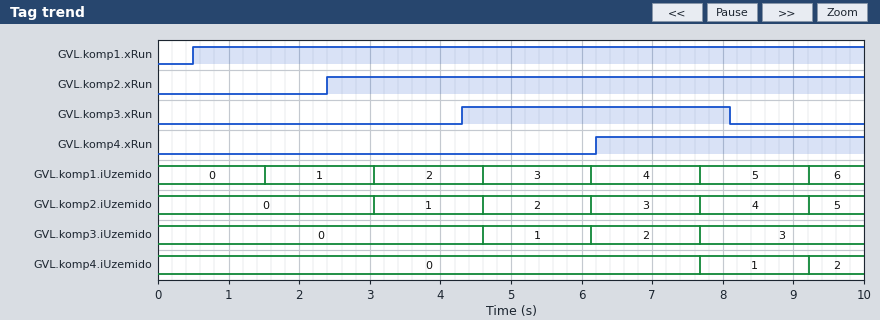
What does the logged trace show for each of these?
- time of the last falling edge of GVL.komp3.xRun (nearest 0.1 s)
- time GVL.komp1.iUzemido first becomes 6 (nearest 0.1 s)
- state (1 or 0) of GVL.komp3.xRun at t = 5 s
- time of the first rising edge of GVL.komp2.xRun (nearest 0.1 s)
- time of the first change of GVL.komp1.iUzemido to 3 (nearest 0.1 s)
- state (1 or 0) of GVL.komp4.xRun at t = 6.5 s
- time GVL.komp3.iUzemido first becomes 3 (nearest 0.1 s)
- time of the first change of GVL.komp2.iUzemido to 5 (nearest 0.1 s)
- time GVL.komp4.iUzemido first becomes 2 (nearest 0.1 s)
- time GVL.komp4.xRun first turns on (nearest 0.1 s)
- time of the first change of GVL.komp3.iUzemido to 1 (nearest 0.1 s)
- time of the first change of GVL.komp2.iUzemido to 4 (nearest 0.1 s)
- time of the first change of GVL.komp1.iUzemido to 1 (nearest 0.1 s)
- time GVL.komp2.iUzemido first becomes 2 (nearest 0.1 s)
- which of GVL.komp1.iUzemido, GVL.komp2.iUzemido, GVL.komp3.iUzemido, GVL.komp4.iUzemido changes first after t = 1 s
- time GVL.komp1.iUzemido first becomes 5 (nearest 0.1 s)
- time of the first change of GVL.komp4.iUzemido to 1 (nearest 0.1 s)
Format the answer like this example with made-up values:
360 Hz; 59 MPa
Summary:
8.1 s; 9.2 s; 1; 2.4 s; 4.6 s; 1; 7.7 s; 9.2 s; 9.2 s; 6.2 s; 4.6 s; 7.7 s; 1.5 s; 4.6 s; GVL.komp1.iUzemido; 7.7 s; 7.7 s
